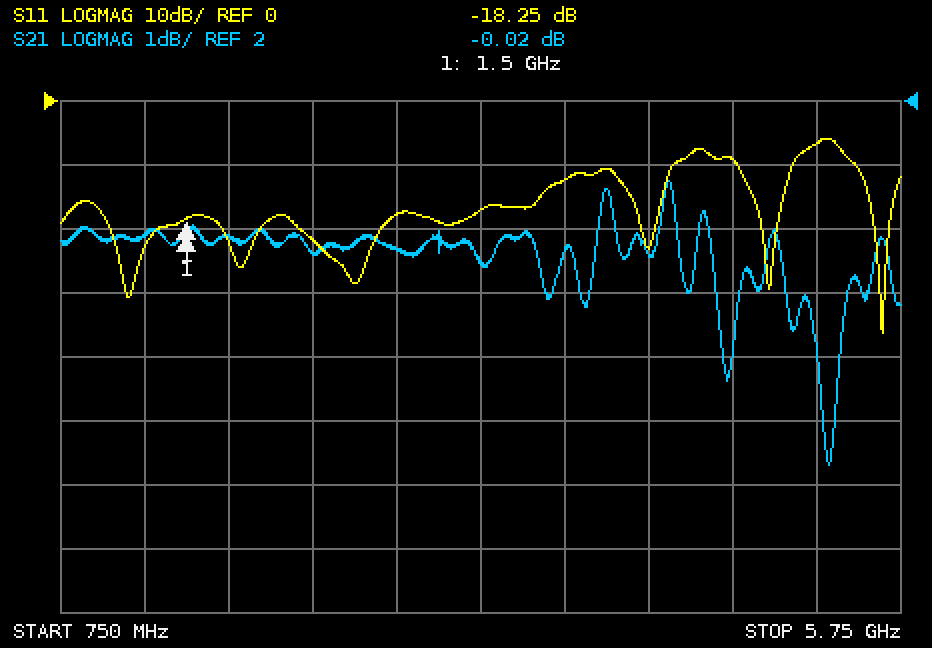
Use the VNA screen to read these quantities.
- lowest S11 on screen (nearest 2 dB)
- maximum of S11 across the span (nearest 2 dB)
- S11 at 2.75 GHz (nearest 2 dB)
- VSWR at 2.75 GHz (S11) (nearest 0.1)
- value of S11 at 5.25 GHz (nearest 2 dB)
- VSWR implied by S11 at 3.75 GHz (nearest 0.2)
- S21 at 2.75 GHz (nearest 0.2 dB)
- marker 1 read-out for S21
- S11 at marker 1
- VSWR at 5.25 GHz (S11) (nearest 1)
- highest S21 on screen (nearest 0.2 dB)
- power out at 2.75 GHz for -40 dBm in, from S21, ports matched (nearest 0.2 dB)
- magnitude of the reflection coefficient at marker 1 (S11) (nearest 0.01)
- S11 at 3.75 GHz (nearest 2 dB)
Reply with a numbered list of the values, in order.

1. -36 dB
2. -6 dB
3. -18 dB
4. 1.3
5. -6 dB
6. 1.6
7. -0.4 dB
8. -0.02 dB
9. -18.25 dB
10. 3
11. 0.8 dB
12. -40.4 dBm
13. 0.12
14. -12 dB
